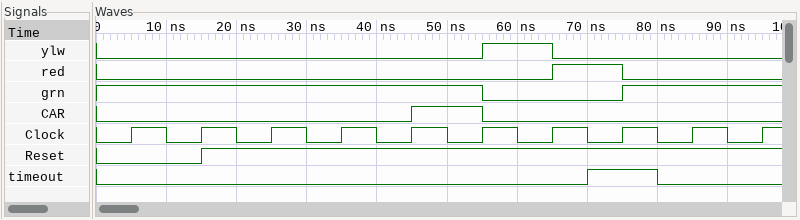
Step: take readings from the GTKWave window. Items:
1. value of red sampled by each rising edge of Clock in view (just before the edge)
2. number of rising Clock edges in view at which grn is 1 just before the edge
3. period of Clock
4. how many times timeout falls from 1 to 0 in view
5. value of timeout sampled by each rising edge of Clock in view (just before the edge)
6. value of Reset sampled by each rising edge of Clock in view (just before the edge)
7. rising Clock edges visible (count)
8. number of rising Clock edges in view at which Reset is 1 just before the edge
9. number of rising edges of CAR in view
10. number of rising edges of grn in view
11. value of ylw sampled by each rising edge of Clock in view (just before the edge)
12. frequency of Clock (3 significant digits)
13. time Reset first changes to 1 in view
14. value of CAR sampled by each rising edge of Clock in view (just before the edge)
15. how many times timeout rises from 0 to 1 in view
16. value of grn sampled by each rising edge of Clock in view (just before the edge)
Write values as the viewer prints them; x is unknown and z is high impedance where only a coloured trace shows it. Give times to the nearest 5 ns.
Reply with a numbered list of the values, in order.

1. 0 0 0 0 0 0 0 1 0 0
2. 8
3. 10 ns
4. 1
5. 0 0 0 0 0 0 0 1 0 0
6. 0 0 1 1 1 1 1 1 1 1
7. 10
8. 8
9. 1
10. 1
11. 0 0 0 0 0 0 1 0 0 0
12. 100 MHz
13. 15 ns
14. 0 0 0 0 0 1 0 0 0 0
15. 1
16. 1 1 1 1 1 1 0 0 1 1
